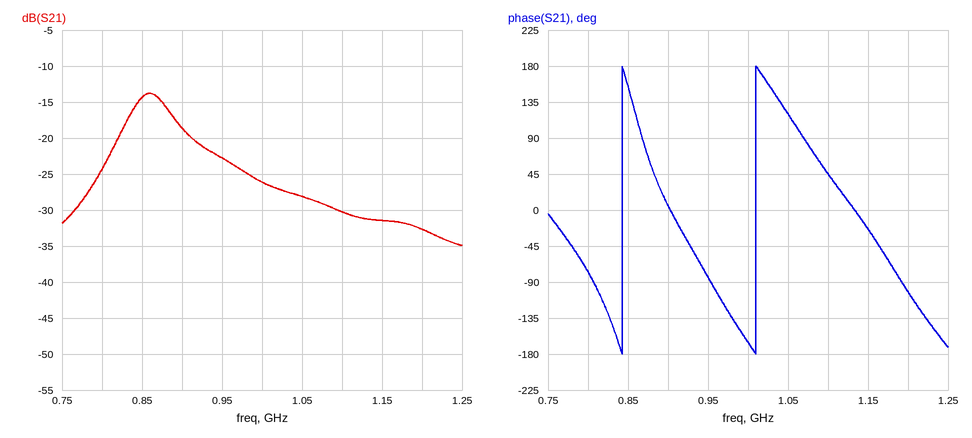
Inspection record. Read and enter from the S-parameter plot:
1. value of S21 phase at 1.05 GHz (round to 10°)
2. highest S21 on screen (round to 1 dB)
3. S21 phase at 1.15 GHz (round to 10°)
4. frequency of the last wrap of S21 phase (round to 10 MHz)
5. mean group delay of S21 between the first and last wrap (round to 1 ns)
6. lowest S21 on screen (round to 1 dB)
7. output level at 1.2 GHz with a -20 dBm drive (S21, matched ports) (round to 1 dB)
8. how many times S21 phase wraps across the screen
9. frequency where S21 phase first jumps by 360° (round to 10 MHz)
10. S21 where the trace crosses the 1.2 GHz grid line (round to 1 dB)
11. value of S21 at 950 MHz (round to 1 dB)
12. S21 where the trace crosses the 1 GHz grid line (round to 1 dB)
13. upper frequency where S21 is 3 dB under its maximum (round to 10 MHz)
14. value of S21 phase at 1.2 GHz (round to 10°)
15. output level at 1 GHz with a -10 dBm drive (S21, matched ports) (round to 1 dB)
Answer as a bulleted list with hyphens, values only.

- 120°
- -14 dB
- -20°
- 1.01 GHz
- 6 ns
- -35 dB
- -53 dBm
- 2
- 840 MHz
- -33 dB
- -23 dB
- -26 dB
- 890 MHz
- -100°
- -36 dBm
